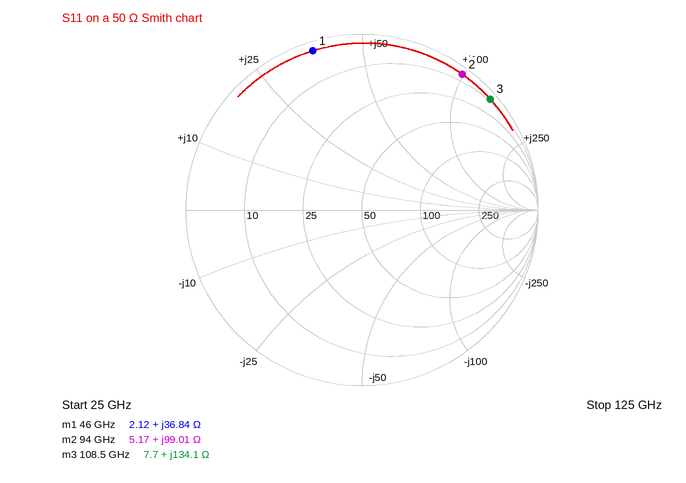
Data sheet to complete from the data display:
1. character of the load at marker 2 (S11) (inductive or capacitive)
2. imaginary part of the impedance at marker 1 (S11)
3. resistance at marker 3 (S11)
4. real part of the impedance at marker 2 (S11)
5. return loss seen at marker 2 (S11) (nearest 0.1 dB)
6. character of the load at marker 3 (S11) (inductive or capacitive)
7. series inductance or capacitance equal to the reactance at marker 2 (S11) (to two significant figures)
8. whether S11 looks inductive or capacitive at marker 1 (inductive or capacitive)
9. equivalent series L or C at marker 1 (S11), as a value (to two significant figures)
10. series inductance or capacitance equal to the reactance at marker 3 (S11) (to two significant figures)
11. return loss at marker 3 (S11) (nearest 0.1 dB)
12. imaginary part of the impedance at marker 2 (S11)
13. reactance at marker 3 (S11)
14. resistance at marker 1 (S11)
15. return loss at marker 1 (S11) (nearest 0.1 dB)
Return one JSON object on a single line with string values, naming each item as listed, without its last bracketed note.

{"character of the load at marker 2 (S11)": "inductive", "imaginary part of the impedance at marker 1": "+36.84 Ω", "resistance at marker 3": "7.7 Ω", "real part of the impedance at marker 2": "5.17 Ω", "return loss seen at marker 2 (S11)": "0.4 dB", "character of the load at marker 3 (S11)": "inductive", "series inductance or capacitance equal to the reactance at marker 2 (S11)": "170 pH", "whether S11 looks inductive or capacitive at marker 1": "inductive", "equivalent series L or C at marker 1 (S11), as a value": "130 pH", "series inductance or capacitance equal to the reactance at marker 3 (S11)": "200 pH", "return loss at marker 3 (S11)": "0.3 dB", "imaginary part of the impedance at marker 2": "+99.01 Ω", "reactance at marker 3": "+134.1 Ω", "resistance at marker 1": "2.12 Ω", "return loss at marker 1 (S11)": "0.5 dB"}
